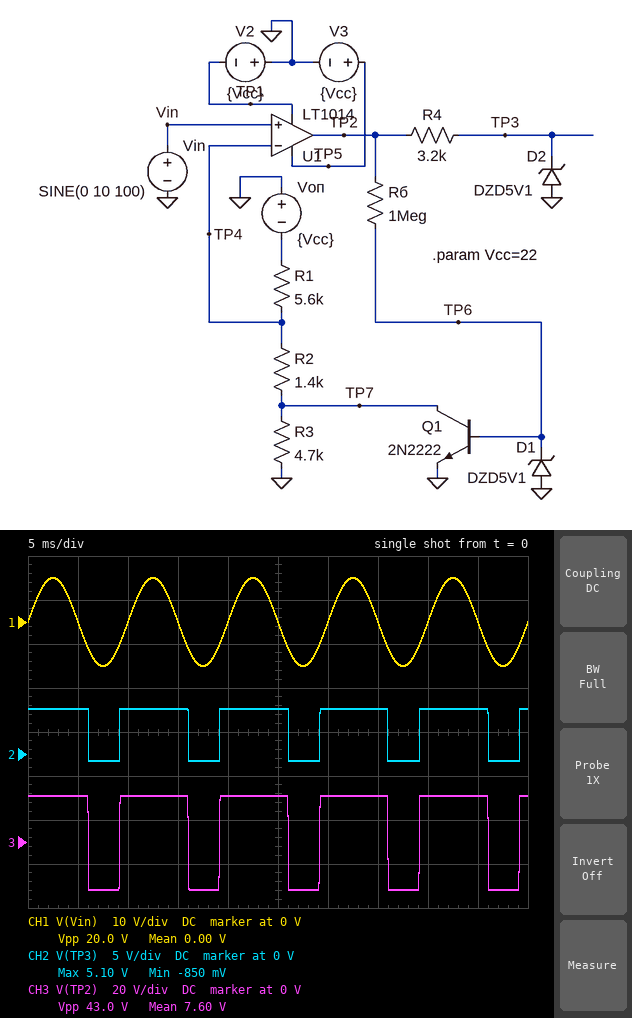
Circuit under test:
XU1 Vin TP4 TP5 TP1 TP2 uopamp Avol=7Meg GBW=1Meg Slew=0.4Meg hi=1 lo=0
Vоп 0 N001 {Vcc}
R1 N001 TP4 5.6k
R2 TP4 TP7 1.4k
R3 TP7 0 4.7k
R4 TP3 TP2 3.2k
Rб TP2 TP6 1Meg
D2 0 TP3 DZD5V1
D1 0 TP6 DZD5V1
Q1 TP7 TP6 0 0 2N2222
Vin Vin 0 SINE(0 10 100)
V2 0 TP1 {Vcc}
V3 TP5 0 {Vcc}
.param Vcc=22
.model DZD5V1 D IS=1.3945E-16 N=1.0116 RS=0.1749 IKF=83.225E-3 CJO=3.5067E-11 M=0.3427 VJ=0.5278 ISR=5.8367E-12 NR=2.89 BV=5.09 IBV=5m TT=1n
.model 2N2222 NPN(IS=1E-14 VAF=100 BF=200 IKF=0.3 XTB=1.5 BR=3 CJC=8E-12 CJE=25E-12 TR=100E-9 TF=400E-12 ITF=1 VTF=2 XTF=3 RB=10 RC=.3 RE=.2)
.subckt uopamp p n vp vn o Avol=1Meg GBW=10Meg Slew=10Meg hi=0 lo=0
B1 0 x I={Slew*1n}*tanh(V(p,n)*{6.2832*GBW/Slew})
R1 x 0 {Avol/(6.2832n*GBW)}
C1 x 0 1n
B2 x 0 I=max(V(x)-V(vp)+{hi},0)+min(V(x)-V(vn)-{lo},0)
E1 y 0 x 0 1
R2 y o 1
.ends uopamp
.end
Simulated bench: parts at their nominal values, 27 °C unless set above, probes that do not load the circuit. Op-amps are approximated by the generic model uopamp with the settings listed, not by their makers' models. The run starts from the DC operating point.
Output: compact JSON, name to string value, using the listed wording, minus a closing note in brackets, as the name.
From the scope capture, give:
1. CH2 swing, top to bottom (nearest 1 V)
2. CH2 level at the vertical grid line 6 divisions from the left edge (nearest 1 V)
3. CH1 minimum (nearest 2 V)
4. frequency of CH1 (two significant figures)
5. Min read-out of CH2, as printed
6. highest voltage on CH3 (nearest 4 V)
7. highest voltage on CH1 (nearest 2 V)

{"CH2 swing, top to bottom": "6 V", "CH2 level at the vertical grid line 6 divisions from the left edge": "5 V", "CH1 minimum": "-10 V", "frequency of CH1": "100 Hz", "Min read-out of CH2, as printed": "-850 mV", "highest voltage on CH3": "20 V", "highest voltage on CH1": "10 V"}
